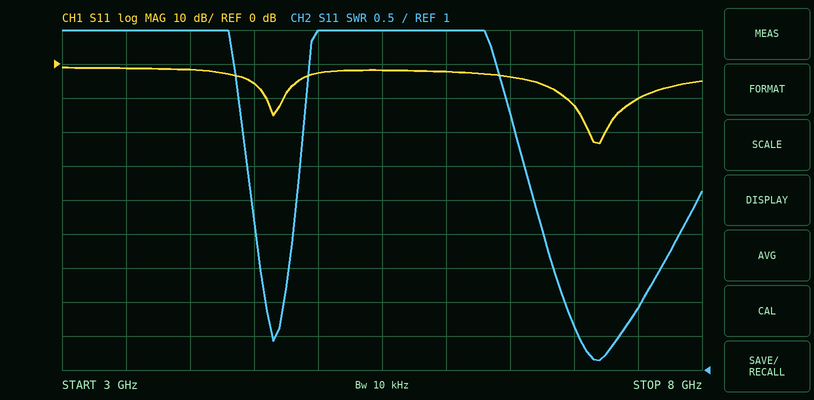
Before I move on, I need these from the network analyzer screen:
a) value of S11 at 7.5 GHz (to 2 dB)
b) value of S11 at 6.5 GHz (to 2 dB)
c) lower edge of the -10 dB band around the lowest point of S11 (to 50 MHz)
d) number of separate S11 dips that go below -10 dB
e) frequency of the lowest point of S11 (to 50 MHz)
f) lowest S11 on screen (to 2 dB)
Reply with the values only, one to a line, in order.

-10 dB
-4 dB
6.95 GHz
2
7.20 GHz
-24 dB
